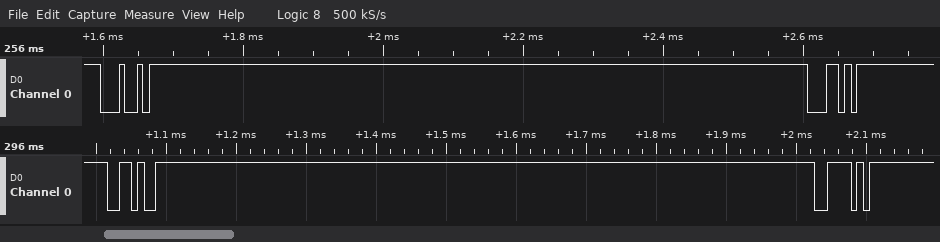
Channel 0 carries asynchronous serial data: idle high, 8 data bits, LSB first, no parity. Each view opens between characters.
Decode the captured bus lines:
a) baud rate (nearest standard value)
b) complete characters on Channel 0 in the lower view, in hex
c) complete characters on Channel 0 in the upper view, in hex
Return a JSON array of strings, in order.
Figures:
["115200 baud", "96, 5E", "A4, AC"]
